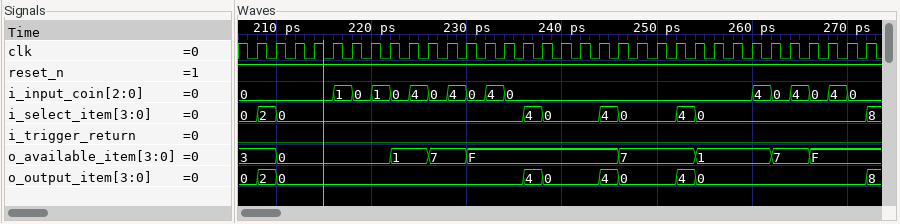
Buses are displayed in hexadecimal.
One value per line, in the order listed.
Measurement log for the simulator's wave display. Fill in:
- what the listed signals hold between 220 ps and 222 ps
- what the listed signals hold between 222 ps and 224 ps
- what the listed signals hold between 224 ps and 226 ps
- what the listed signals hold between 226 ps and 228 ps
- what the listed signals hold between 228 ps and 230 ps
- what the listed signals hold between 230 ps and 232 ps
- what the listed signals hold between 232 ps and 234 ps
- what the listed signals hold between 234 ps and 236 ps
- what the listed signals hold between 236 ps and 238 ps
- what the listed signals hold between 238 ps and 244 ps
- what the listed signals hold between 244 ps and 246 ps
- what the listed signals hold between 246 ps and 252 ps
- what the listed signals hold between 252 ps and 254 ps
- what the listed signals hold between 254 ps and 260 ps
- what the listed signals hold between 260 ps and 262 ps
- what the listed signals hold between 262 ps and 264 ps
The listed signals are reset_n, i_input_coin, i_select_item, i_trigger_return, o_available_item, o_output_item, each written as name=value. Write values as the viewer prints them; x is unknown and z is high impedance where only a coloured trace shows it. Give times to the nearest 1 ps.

reset_n=1, i_input_coin=1, i_select_item=0, i_trigger_return=0, o_available_item=0, o_output_item=0
reset_n=1, i_input_coin=0, i_select_item=0, i_trigger_return=0, o_available_item=1, o_output_item=0
reset_n=1, i_input_coin=4, i_select_item=0, i_trigger_return=0, o_available_item=1, o_output_item=0
reset_n=1, i_input_coin=0, i_select_item=0, i_trigger_return=0, o_available_item=7, o_output_item=0
reset_n=1, i_input_coin=4, i_select_item=0, i_trigger_return=0, o_available_item=7, o_output_item=0
reset_n=1, i_input_coin=0, i_select_item=0, i_trigger_return=0, o_available_item=F, o_output_item=0
reset_n=1, i_input_coin=4, i_select_item=0, i_trigger_return=0, o_available_item=F, o_output_item=0
reset_n=1, i_input_coin=0, i_select_item=0, i_trigger_return=0, o_available_item=F, o_output_item=0
reset_n=1, i_input_coin=0, i_select_item=4, i_trigger_return=0, o_available_item=F, o_output_item=4
reset_n=1, i_input_coin=0, i_select_item=0, i_trigger_return=0, o_available_item=F, o_output_item=0
reset_n=1, i_input_coin=0, i_select_item=4, i_trigger_return=0, o_available_item=F, o_output_item=4
reset_n=1, i_input_coin=0, i_select_item=0, i_trigger_return=0, o_available_item=7, o_output_item=0
reset_n=1, i_input_coin=0, i_select_item=4, i_trigger_return=0, o_available_item=7, o_output_item=4
reset_n=1, i_input_coin=0, i_select_item=0, i_trigger_return=0, o_available_item=1, o_output_item=0
reset_n=1, i_input_coin=4, i_select_item=0, i_trigger_return=0, o_available_item=1, o_output_item=0
reset_n=1, i_input_coin=0, i_select_item=0, i_trigger_return=0, o_available_item=7, o_output_item=0
